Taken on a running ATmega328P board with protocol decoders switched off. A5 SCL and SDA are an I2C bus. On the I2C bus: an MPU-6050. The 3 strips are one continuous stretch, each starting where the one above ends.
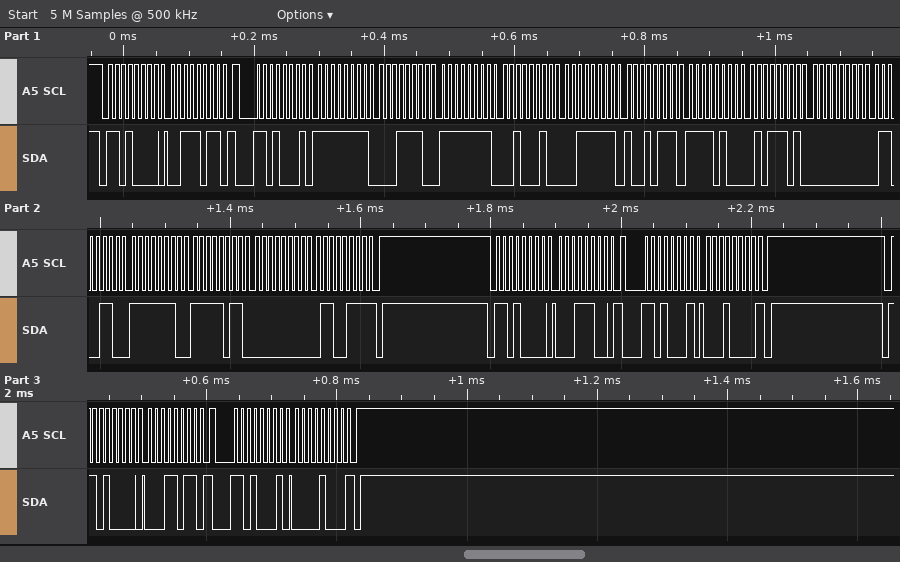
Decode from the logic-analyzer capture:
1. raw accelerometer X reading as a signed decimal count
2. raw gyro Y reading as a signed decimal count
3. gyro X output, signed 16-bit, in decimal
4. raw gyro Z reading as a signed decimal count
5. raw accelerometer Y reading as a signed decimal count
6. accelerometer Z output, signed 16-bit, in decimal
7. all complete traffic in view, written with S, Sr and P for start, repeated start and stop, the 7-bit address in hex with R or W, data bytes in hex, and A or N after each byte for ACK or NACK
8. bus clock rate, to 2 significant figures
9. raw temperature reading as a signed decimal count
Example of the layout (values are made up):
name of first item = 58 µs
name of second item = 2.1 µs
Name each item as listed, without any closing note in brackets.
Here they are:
raw accelerometer X reading as a signed decimal count = -226
raw gyro Y reading as a signed decimal count = -261
gyro X output, signed 16-bit, in decimal = 102
raw gyro Z reading as a signed decimal count = 103
raw accelerometer Y reading as a signed decimal count = -222
accelerometer Z output, signed 16-bit, in decimal = 16279
all complete traffic in view, written with S, Sr and P for start, repeated start and stop, the 7-bit address in hex with R or W, data bytes in hex, and A or N after each byte for ACK or NACK = S 68W A 3B A Sr 68R A FF A 1E A FF A 22 A 3F A 97 A F4 A 5D A 00 A 66 A FE A FB A 00 A 67 N P S 68W A 1C A Sr 68R A 10 N P S 68W A 1B A Sr 68R A 08 N P
bus clock rate, to 2 significant figures = 100 kHz
raw temperature reading as a signed decimal count = -2979
